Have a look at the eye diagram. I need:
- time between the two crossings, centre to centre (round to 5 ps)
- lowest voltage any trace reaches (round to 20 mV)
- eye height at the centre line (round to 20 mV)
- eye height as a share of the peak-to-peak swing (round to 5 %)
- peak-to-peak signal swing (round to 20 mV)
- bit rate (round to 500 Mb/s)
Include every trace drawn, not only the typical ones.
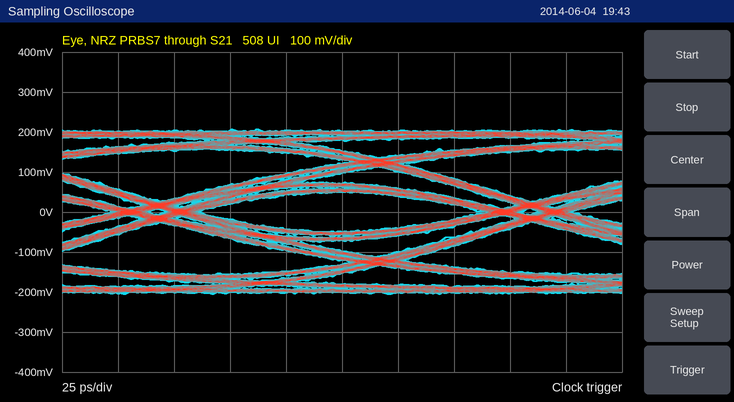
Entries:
165 ps
-200 mV
100 mV
25 %
420 mV
6.0 Gb/s
